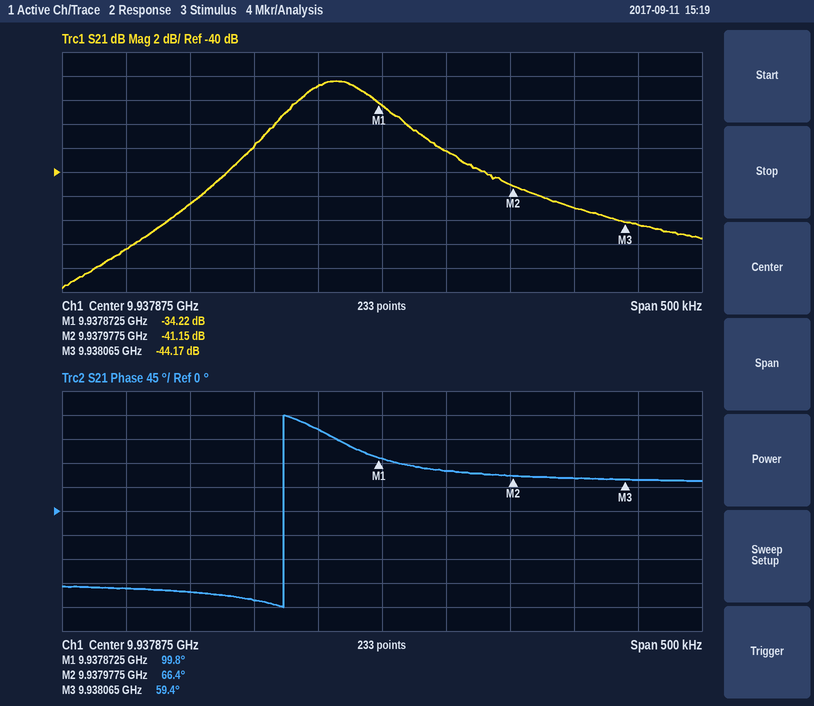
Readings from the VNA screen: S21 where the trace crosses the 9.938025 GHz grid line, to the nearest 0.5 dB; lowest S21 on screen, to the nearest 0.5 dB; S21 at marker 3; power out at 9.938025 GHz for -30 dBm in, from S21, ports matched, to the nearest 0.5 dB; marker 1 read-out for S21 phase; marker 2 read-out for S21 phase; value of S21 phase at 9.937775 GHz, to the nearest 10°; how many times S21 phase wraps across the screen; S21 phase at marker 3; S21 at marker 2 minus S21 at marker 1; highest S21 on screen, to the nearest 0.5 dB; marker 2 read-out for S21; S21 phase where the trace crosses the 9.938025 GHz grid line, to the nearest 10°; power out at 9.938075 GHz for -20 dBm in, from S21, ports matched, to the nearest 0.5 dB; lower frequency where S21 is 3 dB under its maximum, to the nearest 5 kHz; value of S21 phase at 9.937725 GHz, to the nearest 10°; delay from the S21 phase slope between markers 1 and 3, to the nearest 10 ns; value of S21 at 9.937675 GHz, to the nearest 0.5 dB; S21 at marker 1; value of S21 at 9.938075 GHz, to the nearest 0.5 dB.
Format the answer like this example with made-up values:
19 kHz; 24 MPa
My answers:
-43.0 dB; -49.5 dB; -44.17 dB; -73.0 dBm; 99.8°; 66.4°; -170°; 1; 59.4°; -6.93 dB; -32.5 dB; -41.15 dB; 60°; -64.5 dBm; 9.937795 GHz; -150°; 580 ns; -46.5 dB; -34.22 dB; -44.5 dB
